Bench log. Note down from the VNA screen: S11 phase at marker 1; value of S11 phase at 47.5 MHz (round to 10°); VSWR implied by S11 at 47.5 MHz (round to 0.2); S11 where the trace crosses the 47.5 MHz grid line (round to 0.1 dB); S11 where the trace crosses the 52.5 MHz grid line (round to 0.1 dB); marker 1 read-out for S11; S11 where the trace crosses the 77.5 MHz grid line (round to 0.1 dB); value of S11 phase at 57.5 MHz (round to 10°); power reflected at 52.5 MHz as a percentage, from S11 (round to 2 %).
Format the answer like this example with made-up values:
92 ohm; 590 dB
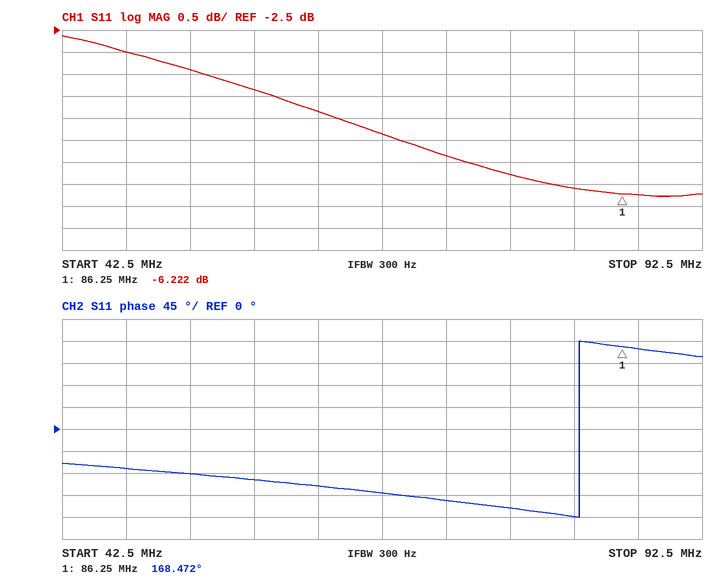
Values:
168.472°; -80°; 5.8; -3.0 dB; -3.4 dB; -6.222 dB; -5.8 dB; -100°; 46 %
